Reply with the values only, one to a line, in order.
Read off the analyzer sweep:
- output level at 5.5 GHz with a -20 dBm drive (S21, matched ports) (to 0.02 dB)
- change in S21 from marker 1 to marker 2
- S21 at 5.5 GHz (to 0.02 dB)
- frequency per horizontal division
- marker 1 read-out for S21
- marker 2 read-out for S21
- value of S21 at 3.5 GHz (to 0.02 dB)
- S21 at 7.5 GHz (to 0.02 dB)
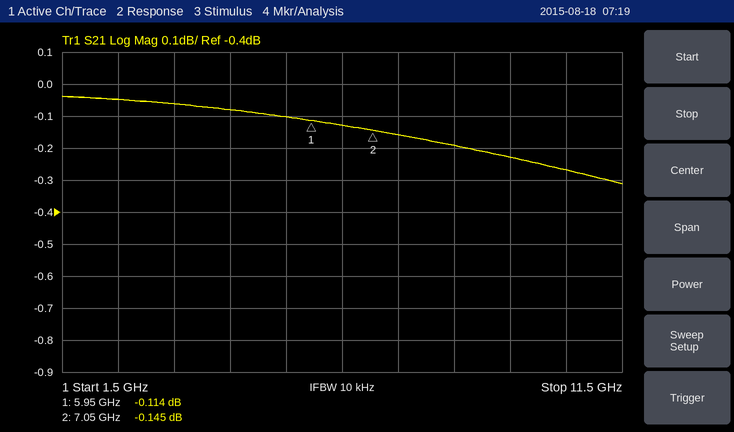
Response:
-20.10 dBm
-0.031 dB
-0.10 dB
1 GHz
-0.114 dB
-0.145 dB
-0.06 dB
-0.16 dB
